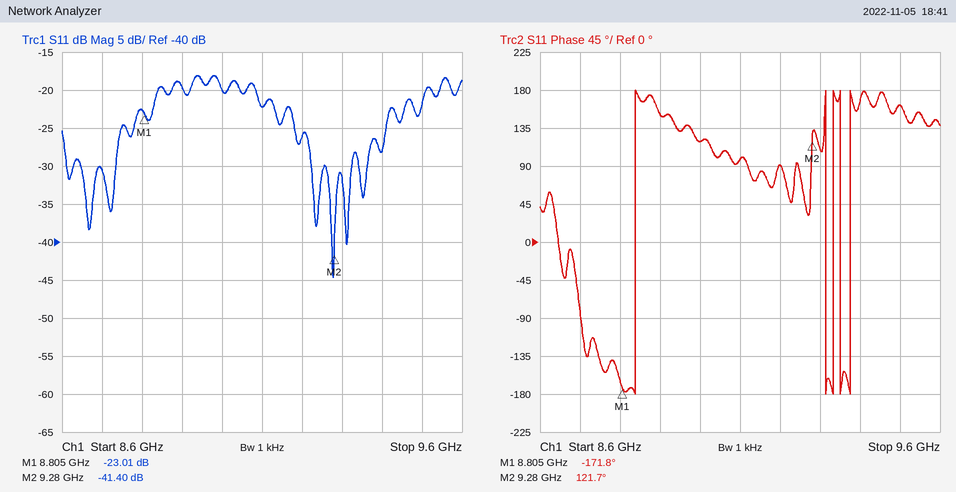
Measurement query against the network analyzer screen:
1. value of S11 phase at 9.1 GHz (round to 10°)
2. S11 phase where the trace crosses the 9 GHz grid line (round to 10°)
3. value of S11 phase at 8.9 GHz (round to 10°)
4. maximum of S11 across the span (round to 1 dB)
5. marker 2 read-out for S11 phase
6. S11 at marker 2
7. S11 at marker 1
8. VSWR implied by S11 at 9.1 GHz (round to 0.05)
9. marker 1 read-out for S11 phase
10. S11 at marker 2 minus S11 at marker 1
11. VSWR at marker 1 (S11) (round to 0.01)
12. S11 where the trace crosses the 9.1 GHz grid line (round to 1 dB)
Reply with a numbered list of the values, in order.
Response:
1. 100°
2. 120°
3. 150°
4. -18 dB
5. 121.7°
6. -41.40 dB
7. -23.01 dB
8. 1.15
9. -171.8°
10. -18.39 dB
11. 1.15
12. -22 dB
